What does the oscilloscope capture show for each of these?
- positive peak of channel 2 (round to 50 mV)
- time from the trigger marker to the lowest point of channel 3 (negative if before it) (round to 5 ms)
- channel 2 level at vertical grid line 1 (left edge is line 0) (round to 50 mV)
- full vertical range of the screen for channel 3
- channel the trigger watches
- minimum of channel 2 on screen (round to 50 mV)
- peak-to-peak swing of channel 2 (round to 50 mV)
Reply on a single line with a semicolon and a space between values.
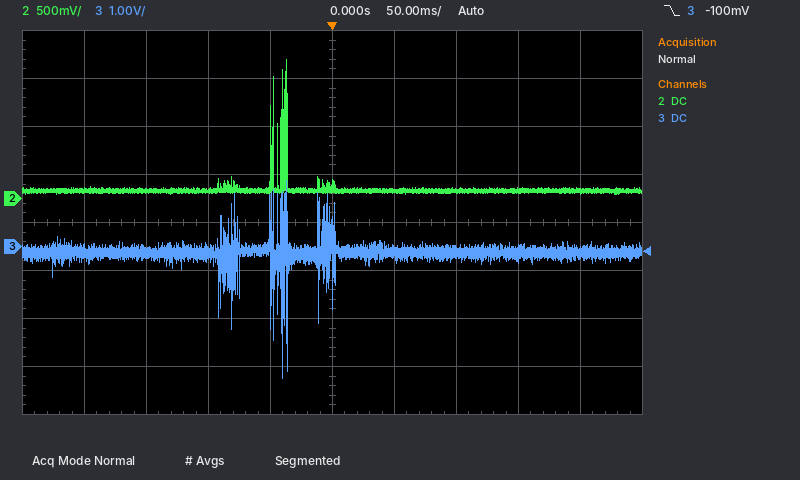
1.45 V; -40 ms; 100 mV; 8 V; channel 3; 50 mV; 1.40 V
